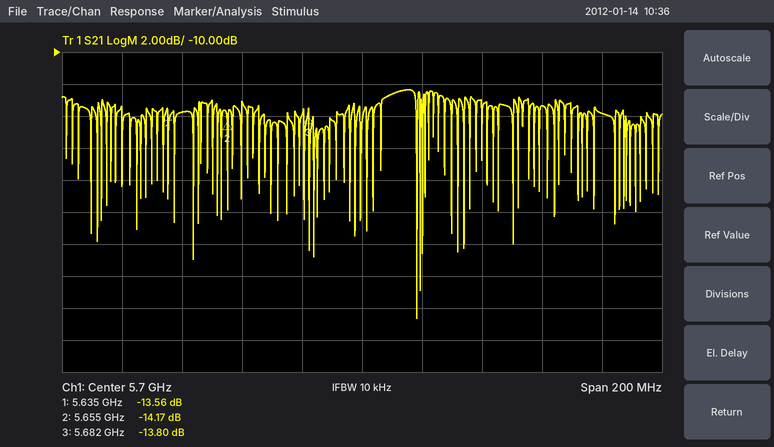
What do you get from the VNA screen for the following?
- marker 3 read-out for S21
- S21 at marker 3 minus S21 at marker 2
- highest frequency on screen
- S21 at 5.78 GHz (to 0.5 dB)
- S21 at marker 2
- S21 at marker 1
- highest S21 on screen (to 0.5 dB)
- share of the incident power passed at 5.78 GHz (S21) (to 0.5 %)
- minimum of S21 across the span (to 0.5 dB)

-13.80 dB
0.37 dB
5.8 GHz
-14.0 dB
-14.17 dB
-13.56 dB
-12.5 dB
4.0 %
-26.5 dB
